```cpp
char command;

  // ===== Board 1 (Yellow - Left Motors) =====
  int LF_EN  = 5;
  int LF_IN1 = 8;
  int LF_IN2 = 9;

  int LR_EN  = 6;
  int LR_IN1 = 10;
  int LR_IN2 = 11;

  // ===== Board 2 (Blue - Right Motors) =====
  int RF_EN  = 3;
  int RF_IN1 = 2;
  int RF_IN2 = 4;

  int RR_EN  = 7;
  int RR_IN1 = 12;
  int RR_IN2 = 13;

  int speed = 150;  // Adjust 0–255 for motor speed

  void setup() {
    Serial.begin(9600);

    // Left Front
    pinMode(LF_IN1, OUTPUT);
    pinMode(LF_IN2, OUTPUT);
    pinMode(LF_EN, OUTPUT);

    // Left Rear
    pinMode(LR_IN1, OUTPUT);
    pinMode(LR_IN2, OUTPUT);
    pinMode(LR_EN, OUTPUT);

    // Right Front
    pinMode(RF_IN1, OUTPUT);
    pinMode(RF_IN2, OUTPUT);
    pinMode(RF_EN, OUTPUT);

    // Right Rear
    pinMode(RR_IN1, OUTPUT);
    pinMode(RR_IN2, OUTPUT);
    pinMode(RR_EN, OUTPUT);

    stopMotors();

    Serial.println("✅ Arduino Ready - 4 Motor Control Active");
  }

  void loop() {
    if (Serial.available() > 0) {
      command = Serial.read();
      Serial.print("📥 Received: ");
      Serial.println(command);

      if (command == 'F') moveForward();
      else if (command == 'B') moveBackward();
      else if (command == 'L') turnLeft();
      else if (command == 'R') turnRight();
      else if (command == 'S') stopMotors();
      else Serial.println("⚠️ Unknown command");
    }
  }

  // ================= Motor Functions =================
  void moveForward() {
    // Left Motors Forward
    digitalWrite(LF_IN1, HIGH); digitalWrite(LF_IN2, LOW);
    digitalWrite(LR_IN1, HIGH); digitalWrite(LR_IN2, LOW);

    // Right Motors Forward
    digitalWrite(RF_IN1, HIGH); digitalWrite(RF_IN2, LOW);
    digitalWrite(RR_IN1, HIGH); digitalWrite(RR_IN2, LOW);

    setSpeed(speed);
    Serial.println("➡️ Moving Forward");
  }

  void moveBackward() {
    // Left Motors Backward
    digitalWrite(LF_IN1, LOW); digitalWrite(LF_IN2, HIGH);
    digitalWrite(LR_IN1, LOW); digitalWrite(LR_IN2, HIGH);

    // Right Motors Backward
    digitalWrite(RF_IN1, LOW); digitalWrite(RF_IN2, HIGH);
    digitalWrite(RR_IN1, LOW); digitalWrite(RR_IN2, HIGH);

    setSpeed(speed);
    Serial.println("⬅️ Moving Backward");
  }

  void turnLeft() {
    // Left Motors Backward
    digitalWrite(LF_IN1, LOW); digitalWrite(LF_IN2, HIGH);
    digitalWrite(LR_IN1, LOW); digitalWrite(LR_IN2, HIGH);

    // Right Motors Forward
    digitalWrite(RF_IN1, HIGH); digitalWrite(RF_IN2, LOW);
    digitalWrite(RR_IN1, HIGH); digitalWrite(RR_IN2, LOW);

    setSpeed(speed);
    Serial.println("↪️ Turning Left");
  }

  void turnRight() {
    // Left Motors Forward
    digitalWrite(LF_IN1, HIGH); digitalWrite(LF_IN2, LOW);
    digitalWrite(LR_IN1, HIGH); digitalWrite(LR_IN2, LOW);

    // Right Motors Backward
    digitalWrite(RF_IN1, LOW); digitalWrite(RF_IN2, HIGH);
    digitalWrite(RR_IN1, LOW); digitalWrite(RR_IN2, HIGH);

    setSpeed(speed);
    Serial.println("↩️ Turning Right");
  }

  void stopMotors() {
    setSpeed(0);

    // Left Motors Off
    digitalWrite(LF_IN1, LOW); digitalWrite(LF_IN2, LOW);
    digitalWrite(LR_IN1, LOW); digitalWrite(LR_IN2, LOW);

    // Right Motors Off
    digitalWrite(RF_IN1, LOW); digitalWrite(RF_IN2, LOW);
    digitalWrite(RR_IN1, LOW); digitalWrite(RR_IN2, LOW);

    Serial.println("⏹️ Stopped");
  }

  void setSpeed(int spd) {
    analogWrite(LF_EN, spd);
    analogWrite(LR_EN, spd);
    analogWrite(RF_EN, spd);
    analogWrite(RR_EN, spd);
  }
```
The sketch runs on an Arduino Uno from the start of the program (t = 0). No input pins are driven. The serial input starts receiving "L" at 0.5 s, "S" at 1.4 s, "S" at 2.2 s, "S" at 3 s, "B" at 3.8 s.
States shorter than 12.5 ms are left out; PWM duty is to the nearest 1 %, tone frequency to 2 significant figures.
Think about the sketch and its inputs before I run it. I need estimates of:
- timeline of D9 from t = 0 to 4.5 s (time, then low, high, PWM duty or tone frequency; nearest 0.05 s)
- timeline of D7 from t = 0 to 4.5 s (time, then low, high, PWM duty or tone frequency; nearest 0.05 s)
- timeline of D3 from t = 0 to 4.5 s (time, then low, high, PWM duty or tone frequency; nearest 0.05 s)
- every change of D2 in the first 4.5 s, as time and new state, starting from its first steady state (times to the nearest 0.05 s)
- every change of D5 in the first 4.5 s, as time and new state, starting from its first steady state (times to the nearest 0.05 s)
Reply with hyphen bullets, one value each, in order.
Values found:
- 0 s low; 0.5 s high; 1.4 s low; 3.8 s high
- 0 s low; 0.5 s high; 1.4 s low; 3.8 s high
- 0 s low; 0.5 s PWM 59 %; 1.4 s low; 3.8 s PWM 59 %
- 0 s low; 0.5 s high; 1.4 s low
- 0 s low; 0.5 s PWM 59 %; 1.4 s low; 3.8 s PWM 59 %
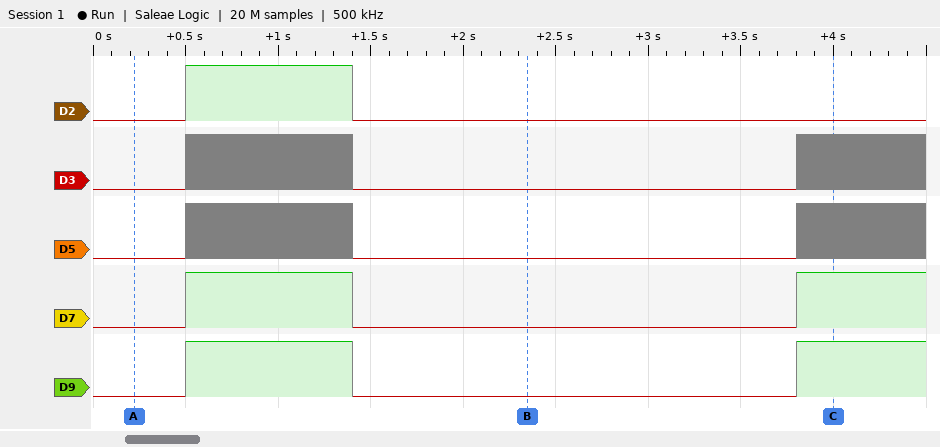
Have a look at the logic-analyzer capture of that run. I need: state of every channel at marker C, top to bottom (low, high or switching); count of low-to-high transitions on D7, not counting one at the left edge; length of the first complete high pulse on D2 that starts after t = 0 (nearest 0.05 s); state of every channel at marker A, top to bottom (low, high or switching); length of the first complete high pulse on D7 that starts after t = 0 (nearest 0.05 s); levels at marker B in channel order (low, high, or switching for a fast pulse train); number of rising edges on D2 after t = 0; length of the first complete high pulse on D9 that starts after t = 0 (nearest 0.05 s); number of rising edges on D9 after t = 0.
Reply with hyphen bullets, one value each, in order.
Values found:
- D2 low, D3 switching, D5 switching, D7 high, D9 high
- 2
- 0.90 s
- D2 low, D3 low, D5 low, D7 low, D9 low
- 0.90 s
- D2 low, D3 low, D5 low, D7 low, D9 low
- 1
- 0.90 s
- 2
